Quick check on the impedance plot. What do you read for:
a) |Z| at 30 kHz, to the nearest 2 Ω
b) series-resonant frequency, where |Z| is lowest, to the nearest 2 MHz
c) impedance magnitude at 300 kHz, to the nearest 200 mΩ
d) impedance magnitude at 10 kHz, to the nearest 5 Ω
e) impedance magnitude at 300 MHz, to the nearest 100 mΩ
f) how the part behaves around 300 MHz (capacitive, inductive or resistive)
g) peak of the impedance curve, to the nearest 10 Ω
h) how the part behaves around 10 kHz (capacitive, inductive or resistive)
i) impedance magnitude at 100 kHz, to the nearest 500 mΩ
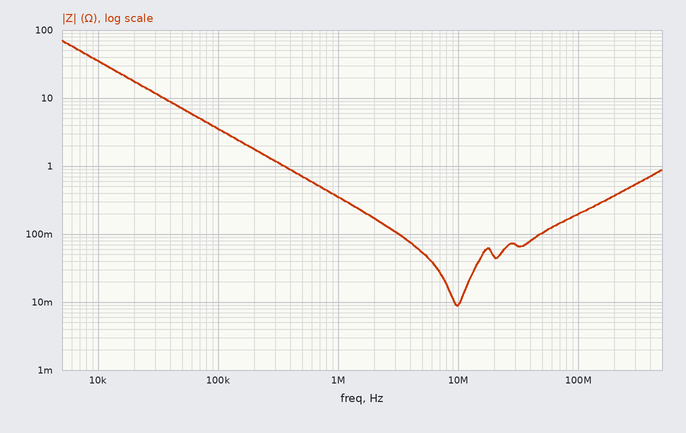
12 Ω
10 MHz
1.2 Ω
35 Ω
500 mΩ
inductive
70 Ω
capacitive
3.5 Ω
